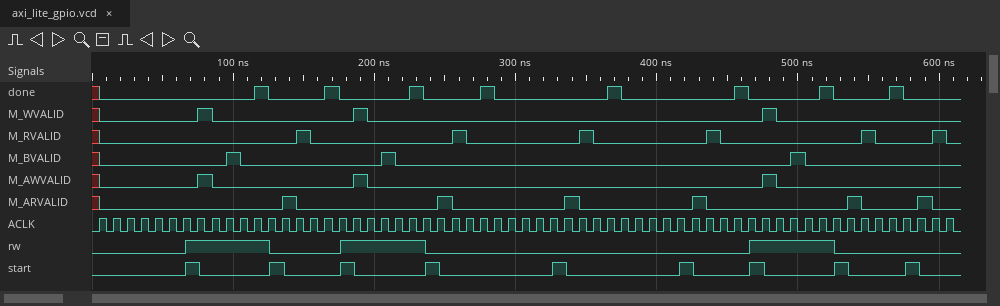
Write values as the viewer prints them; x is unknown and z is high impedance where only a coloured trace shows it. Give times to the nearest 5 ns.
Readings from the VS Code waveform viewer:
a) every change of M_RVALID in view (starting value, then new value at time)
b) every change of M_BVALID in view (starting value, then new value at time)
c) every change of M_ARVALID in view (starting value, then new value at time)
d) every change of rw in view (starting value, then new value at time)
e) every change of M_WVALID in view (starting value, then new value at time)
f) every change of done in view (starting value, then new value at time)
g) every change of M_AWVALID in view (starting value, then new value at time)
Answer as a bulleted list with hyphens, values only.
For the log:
- x, 0 at 5 ns, 1 at 145 ns, 0 at 155 ns, 1 at 255 ns, 0 at 265 ns, 1 at 345 ns, 0 at 355 ns, 1 at 435 ns, 0 at 445 ns, 1 at 545 ns, 0 at 555 ns, 1 at 595 ns, 0 at 605 ns
- x, 0 at 5 ns, 1 at 95 ns, 0 at 105 ns, 1 at 205 ns, 0 at 215 ns, 1 at 495 ns, 0 at 505 ns
- x, 0 at 5 ns, 1 at 135 ns, 0 at 145 ns, 1 at 245 ns, 0 at 255 ns, 1 at 335 ns, 0 at 345 ns, 1 at 425 ns, 0 at 435 ns, 1 at 535 ns, 0 at 545 ns, 1 at 585 ns, 0 at 595 ns
- 0, 1 at 65 ns, 0 at 125 ns, 1 at 175 ns, 0 at 235 ns, 1 at 465 ns, 0 at 525 ns
- x, 0 at 5 ns, 1 at 75 ns, 0 at 85 ns, 1 at 185 ns, 0 at 195 ns, 1 at 475 ns, 0 at 485 ns
- x, 0 at 5 ns, 1 at 115 ns, 0 at 125 ns, 1 at 165 ns, 0 at 175 ns, 1 at 225 ns, 0 at 235 ns, 1 at 275 ns, 0 at 285 ns, 1 at 365 ns, 0 at 375 ns, 1 at 455 ns, 0 at 465 ns, 1 at 515 ns, 0 at 525 ns, 1 at 565 ns, 0 at 575 ns
- x, 0 at 5 ns, 1 at 75 ns, 0 at 85 ns, 1 at 185 ns, 0 at 195 ns, 1 at 475 ns, 0 at 485 ns
